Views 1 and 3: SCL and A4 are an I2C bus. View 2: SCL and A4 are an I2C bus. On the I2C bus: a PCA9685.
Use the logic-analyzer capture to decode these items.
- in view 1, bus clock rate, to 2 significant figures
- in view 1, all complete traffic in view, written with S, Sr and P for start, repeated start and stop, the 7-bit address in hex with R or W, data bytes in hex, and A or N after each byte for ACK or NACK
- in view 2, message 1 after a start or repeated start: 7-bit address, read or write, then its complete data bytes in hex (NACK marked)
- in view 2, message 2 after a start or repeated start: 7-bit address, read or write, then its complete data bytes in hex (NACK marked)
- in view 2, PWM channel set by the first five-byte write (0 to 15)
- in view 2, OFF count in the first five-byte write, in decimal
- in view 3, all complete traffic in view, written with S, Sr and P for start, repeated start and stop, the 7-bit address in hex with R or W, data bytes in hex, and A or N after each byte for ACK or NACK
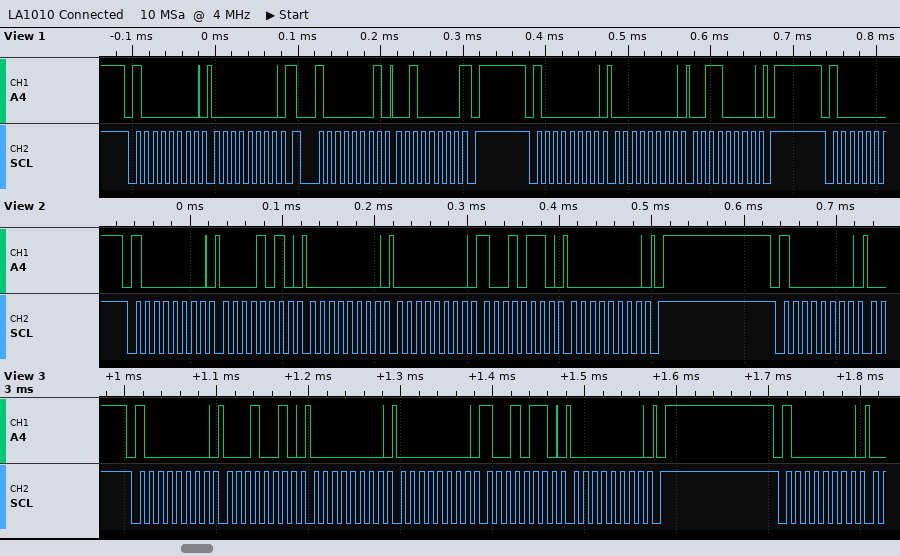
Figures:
100 kHz
S 40W A 00 A Sr 40R A 20 N P S 40W A 00 A 30 A P
0x40 write: 0A 00 00 96 00
0x40 write
1
150
S 40W A 12 A 00 A 00 A 96 A 00 A P S 40W A
